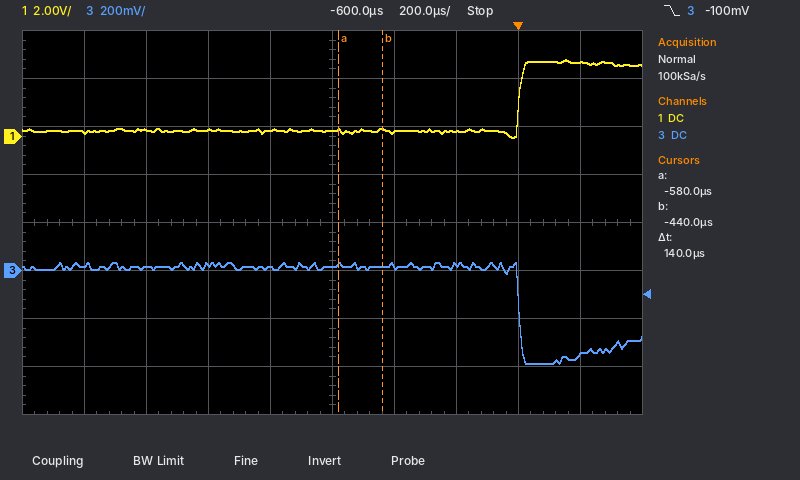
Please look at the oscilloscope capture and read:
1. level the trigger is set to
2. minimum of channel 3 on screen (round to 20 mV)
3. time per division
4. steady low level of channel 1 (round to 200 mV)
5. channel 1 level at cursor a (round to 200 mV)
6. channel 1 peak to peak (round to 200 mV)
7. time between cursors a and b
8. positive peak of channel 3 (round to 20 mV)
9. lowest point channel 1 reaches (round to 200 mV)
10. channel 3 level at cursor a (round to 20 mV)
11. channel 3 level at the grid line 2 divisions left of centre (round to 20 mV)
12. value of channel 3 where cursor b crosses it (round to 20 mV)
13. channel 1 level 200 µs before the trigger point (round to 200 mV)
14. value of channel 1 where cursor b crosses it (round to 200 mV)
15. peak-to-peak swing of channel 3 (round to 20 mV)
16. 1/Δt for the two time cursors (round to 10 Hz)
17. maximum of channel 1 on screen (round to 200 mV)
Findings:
-100 mV
-380 mV
200 µs
200 mV
200 mV
3.2 V
140 µs
40 mV
0.0 V
20 mV
20 mV
20 mV
200 mV
200 mV
420 mV
7.14 kHz
3.2 V
